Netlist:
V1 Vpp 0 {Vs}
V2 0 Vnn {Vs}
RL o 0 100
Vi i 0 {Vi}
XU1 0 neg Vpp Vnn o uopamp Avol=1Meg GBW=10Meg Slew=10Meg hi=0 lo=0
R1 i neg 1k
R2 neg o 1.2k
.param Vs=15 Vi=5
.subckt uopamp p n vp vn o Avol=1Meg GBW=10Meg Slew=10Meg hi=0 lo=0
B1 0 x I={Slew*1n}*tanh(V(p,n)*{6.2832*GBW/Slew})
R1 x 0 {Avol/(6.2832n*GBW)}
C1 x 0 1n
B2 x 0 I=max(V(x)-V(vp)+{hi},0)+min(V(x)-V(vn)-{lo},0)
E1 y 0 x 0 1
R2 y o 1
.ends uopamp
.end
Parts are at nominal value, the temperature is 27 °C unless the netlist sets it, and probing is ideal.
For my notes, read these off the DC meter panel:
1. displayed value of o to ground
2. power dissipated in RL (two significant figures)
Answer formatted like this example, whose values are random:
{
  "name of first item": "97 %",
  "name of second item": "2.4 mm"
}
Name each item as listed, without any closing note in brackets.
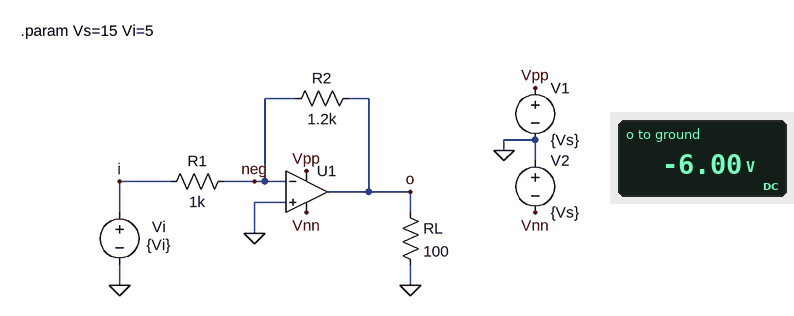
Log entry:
{
  "displayed value of o to ground": "-6.00 V",
  "power dissipated in RL": "360 mW"
}
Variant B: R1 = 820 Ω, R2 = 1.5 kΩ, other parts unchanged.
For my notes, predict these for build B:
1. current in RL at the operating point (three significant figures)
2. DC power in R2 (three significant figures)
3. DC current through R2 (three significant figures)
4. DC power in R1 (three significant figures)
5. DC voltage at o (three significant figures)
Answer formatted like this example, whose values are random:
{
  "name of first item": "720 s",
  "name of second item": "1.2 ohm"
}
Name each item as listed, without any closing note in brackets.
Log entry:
{
  "current in RL at the operating point": "91.5 mA",
  "DC power in R2": "55.8 mW",
  "DC current through R2": "6.10 mA",
  "DC power in R1": "30.5 mW",
  "DC voltage at o": "-9.15 V"
}
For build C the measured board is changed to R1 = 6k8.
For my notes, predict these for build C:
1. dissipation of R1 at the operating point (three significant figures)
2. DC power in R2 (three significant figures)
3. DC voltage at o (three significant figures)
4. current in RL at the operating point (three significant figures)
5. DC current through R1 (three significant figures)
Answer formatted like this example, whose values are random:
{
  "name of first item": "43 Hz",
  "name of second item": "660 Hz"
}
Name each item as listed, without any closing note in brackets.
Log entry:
{
  "dissipation of R1 at the operating point": "3.68 mW",
  "DC power in R2": "649 µW",
  "DC voltage at o": "-882 mV",
  "current in RL at the operating point": "8.82 mA",
  "DC current through R1": "735 µA"
}
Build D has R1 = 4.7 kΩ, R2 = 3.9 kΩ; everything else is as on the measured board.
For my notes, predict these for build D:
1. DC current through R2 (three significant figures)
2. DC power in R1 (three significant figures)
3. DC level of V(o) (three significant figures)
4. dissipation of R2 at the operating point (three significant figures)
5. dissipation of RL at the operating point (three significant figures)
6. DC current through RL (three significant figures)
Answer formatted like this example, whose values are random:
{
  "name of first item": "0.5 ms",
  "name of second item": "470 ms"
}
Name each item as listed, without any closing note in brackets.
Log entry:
{
  "DC current through R2": "1.06 mA",
  "DC power in R1": "5.32 mW",
  "DC level of V(o)": "-4.15 V",
  "dissipation of R2 at the operating point": "4.41 mW",
  "dissipation of RL at the operating point": "172 mW",
  "DC current through RL": "41.5 mA"
}
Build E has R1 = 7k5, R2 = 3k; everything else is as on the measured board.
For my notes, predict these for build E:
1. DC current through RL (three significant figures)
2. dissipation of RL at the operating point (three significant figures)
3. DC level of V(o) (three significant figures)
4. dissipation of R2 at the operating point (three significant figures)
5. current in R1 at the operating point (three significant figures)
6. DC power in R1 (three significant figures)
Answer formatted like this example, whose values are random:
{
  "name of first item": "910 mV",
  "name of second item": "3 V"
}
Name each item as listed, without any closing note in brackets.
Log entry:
{
  "DC current through RL": "20.0 mA",
  "dissipation of RL at the operating point": "40.0 mW",
  "DC level of V(o)": "-2.00 V",
  "dissipation of R2 at the operating point": "1.33 mW",
  "current in R1 at the operating point": "667 µA",
  "DC power in R1": "3.33 mW"
}
